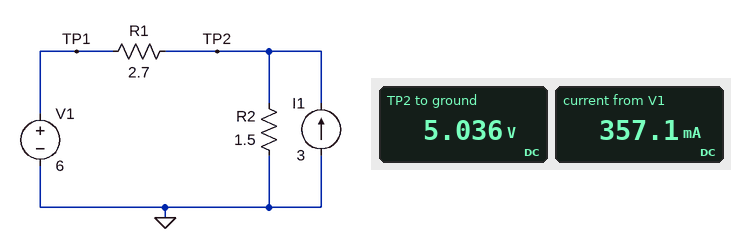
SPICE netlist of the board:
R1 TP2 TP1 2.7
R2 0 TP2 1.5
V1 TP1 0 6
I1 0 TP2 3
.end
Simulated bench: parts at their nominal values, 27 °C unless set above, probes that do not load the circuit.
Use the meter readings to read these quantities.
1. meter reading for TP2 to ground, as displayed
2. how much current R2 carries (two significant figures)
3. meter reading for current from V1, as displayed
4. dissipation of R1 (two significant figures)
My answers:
5.036 V
3.4 A
357.1 mA
340 mW
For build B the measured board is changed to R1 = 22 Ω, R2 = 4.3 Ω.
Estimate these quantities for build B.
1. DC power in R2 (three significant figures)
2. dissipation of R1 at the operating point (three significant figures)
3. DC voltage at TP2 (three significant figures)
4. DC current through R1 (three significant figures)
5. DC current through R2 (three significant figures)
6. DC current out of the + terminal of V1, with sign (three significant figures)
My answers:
32.2 W
1.51 W
11.8 V
262 mA
2.74 A
-262 mA
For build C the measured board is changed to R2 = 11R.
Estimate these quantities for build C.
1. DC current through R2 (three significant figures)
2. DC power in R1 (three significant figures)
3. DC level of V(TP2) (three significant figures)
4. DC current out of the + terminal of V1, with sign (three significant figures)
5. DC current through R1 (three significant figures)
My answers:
1.03 A
10.5 W
11.3 V
-1.97 A
1.97 A
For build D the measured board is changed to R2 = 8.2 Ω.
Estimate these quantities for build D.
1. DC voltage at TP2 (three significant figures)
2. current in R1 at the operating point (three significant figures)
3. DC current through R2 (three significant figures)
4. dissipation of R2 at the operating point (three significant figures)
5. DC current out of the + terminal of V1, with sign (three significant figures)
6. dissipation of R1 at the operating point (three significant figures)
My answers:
10.6 V
1.71 A
1.29 A
13.7 W
-1.71 A
7.86 W
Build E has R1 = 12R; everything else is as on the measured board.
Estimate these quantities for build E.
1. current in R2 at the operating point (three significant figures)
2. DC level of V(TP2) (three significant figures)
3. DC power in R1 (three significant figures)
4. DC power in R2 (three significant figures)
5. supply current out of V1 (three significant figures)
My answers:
3.11 A
4.67 V
148 mW
14.5 W
111 mA
